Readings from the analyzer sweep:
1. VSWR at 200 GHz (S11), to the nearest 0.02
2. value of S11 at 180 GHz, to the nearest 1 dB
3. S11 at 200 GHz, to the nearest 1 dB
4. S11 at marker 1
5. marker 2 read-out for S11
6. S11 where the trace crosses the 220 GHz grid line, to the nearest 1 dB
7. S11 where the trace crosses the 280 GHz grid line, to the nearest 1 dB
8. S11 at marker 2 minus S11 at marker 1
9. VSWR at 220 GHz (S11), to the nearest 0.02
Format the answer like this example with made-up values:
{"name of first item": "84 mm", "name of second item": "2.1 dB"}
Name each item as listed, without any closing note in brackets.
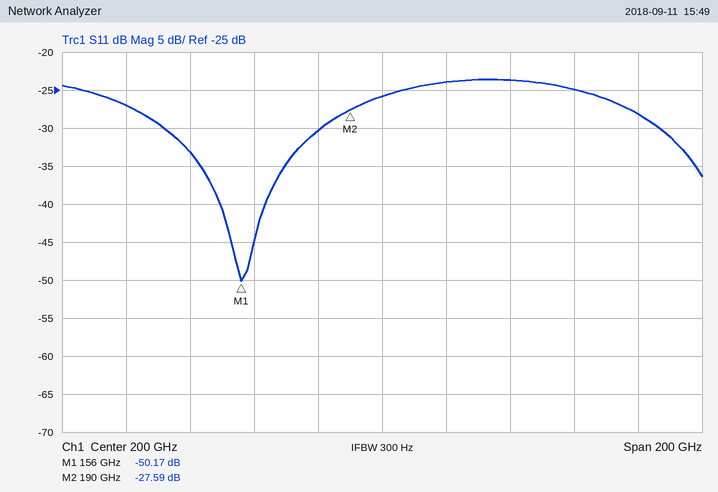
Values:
{"VSWR at 200 GHz (S11), to the nearest 0.02": "1.10", "value of S11 at 180 GHz, to the nearest 1 dB": "-30 dB", "S11 at 200 GHz, to the nearest 1 dB": "-26 dB", "S11 at marker 1": "-50.17 dB", "marker 2 read-out for S11": "-27.59 dB", "S11 where the trace crosses the 220 GHz grid line, to the nearest 1 dB": "-24 dB", "S11 where the trace crosses the 280 GHz grid line, to the nearest 1 dB": "-28 dB", "S11 at marker 2 minus S11 at marker 1": "22.58 dB", "VSWR at 220 GHz (S11), to the nearest 0.02": "1.14"}
